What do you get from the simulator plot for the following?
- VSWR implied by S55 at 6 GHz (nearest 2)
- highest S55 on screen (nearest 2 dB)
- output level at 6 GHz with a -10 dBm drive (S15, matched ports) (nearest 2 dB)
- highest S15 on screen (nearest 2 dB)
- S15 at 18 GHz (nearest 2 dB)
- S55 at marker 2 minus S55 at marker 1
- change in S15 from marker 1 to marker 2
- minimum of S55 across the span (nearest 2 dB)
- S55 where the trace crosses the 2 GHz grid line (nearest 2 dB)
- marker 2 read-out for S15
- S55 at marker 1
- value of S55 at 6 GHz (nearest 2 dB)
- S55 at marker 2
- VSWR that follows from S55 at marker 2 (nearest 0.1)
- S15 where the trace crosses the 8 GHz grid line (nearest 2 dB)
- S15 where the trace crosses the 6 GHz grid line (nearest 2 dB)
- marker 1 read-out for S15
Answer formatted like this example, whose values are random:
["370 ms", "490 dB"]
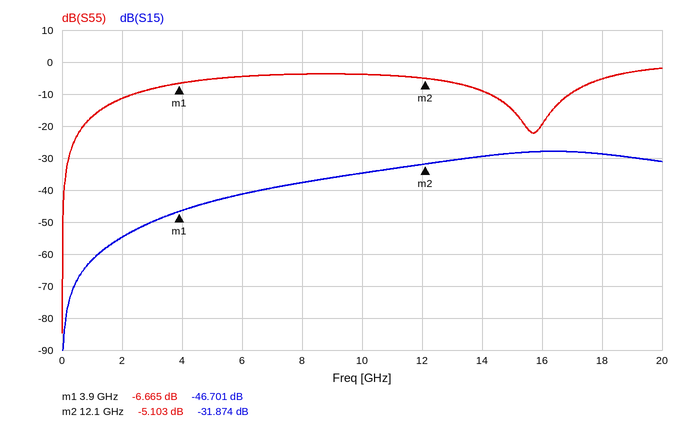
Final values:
["4", "-2 dB", "-52 dBm", "-28 dB", "-28 dB", "1.562 dB", "14.827 dB", "-84 dB", "-12 dB", "-31.874 dB", "-6.665 dB", "-4 dB", "-5.103 dB", "3.5", "-38 dB", "-42 dB", "-46.701 dB"]
